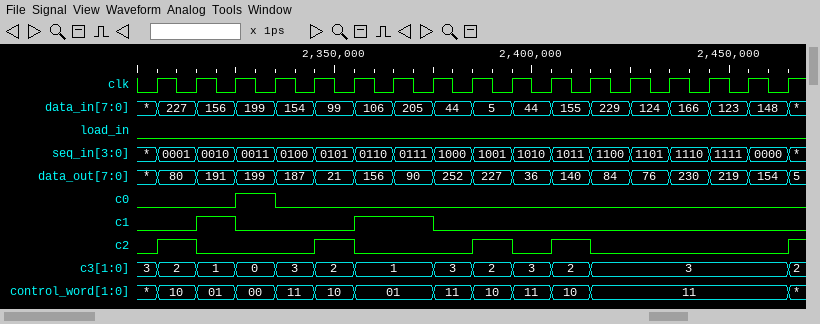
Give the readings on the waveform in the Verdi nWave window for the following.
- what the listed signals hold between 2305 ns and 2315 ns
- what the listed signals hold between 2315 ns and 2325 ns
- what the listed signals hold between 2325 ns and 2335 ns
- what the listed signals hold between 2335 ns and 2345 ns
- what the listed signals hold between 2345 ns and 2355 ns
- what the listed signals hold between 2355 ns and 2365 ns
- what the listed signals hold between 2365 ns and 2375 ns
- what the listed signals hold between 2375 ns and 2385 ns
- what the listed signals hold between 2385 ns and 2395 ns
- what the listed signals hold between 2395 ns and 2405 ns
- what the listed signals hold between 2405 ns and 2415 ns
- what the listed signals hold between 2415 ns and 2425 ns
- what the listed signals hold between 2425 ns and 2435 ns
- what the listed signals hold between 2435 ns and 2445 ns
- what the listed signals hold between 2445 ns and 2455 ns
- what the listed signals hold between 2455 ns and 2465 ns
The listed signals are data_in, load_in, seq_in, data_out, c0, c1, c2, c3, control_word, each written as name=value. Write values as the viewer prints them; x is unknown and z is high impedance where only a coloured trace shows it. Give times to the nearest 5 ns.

data_in=227, load_in=0, seq_in=0001, data_out=80, c0=0, c1=0, c2=1, c3=2, control_word=10
data_in=156, load_in=0, seq_in=0010, data_out=191, c0=0, c1=1, c2=0, c3=1, control_word=01
data_in=199, load_in=0, seq_in=0011, data_out=199, c0=1, c1=0, c2=0, c3=0, control_word=00
data_in=154, load_in=0, seq_in=0100, data_out=187, c0=0, c1=0, c2=0, c3=3, control_word=11
data_in=99, load_in=0, seq_in=0101, data_out=21, c0=0, c1=0, c2=1, c3=2, control_word=10
data_in=106, load_in=0, seq_in=0110, data_out=156, c0=0, c1=1, c2=0, c3=1, control_word=01
data_in=205, load_in=0, seq_in=0111, data_out=90, c0=0, c1=1, c2=0, c3=1, control_word=01
data_in=44, load_in=0, seq_in=1000, data_out=252, c0=0, c1=0, c2=0, c3=3, control_word=11
data_in=5, load_in=0, seq_in=1001, data_out=227, c0=0, c1=0, c2=1, c3=2, control_word=10
data_in=44, load_in=0, seq_in=1010, data_out=36, c0=0, c1=0, c2=0, c3=3, control_word=11
data_in=155, load_in=0, seq_in=1011, data_out=140, c0=0, c1=0, c2=1, c3=2, control_word=10
data_in=229, load_in=0, seq_in=1100, data_out=84, c0=0, c1=0, c2=0, c3=3, control_word=11
data_in=124, load_in=0, seq_in=1101, data_out=76, c0=0, c1=0, c2=0, c3=3, control_word=11
data_in=166, load_in=0, seq_in=1110, data_out=230, c0=0, c1=0, c2=0, c3=3, control_word=11
data_in=123, load_in=0, seq_in=1111, data_out=219, c0=0, c1=0, c2=0, c3=3, control_word=11
data_in=148, load_in=0, seq_in=0000, data_out=154, c0=0, c1=0, c2=0, c3=3, control_word=11
